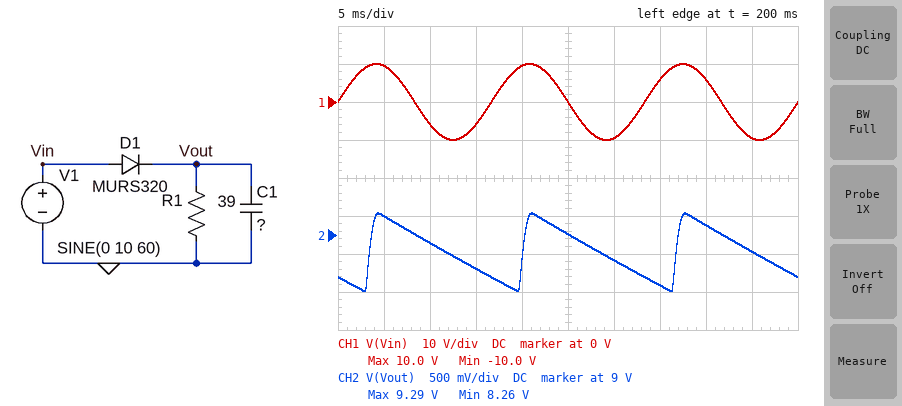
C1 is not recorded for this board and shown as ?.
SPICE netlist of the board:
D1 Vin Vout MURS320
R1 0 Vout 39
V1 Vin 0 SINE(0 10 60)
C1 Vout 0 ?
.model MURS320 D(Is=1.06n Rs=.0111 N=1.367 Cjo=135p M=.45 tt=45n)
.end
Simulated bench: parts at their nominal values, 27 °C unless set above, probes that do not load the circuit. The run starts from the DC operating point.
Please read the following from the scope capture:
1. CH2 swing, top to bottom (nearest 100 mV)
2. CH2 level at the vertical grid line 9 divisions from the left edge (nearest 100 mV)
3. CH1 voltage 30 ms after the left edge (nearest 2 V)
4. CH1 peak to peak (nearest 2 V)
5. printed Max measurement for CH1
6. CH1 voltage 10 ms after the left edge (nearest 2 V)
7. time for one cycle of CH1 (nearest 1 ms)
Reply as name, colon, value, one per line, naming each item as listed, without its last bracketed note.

CH2 swing, top to bottom: 1.0 V
CH2 level at the vertical grid line 9 divisions from the left edge: 8.8 V
CH1 voltage 30 ms after the left edge: -10 V
CH1 peak to peak: 20 V
printed Max measurement for CH1: 10.0 V
CH1 voltage 10 ms after the left edge: -6 V
time for one cycle of CH1: 17 ms
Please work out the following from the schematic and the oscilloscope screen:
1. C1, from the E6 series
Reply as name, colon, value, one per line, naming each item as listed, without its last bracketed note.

C1, from the E6 series: 3.3 mF
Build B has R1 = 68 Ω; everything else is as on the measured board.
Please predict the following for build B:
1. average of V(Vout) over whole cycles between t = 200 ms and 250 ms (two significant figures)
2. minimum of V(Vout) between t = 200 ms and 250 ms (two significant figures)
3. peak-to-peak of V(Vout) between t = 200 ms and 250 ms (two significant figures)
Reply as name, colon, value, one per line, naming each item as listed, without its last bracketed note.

average of V(Vout) over whole cycles between t = 200 ms and 250 ms: 9.0 V
minimum of V(Vout) between t = 200 ms and 250 ms: 8.7 V
peak-to-peak of V(Vout) between t = 200 ms and 250 ms: 610 mV
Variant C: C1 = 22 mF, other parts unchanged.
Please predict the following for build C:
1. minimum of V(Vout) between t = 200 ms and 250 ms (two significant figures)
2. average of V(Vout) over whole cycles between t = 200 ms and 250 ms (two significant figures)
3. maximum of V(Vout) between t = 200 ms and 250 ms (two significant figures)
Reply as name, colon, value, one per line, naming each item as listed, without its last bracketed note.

minimum of V(Vout) between t = 200 ms and 250 ms: 9.0 V
average of V(Vout) over whole cycles between t = 200 ms and 250 ms: 9.1 V
maximum of V(Vout) between t = 200 ms and 250 ms: 9.2 V
